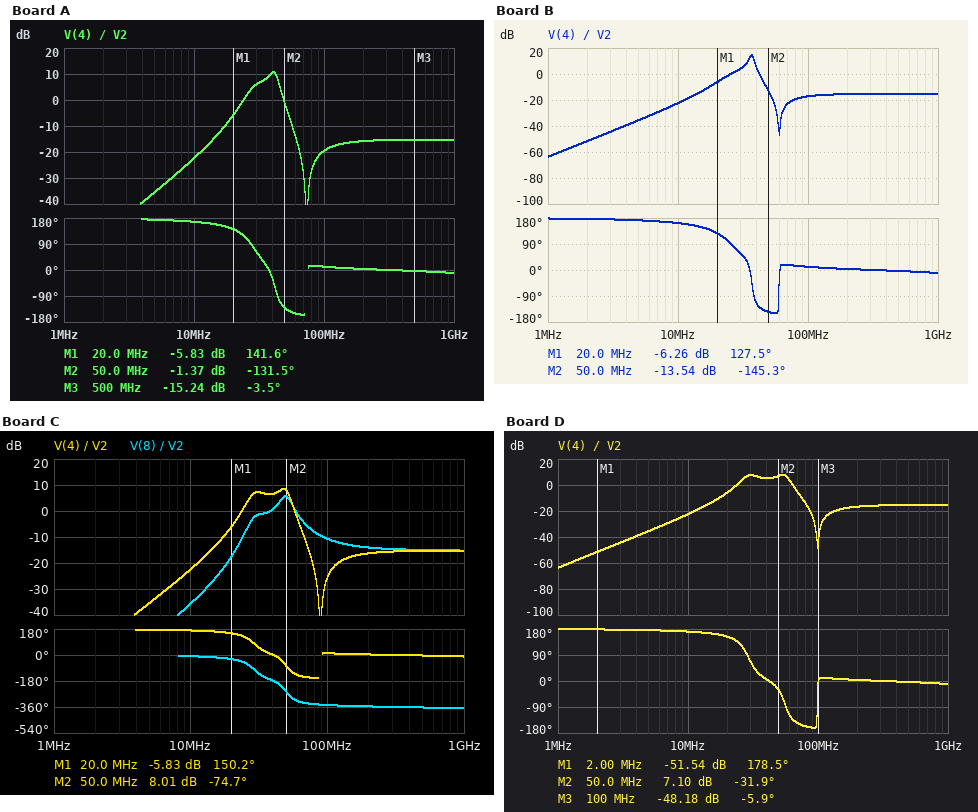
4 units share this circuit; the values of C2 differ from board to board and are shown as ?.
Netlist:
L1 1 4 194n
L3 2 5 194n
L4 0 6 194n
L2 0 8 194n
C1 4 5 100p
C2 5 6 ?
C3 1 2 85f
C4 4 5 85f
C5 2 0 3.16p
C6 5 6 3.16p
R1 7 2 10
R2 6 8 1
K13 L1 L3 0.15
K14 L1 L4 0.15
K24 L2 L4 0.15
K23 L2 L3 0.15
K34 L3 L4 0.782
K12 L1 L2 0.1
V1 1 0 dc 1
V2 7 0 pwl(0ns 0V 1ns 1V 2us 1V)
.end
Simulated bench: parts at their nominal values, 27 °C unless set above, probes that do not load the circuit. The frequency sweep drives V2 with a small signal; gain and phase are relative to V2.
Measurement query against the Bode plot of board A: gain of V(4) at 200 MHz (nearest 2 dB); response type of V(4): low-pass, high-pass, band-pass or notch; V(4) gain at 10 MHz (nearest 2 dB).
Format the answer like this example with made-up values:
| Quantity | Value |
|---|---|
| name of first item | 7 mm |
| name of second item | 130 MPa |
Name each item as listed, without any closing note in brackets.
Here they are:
| Quantity | Value |
|---|---|
| gain of V(4) at 200 MHz | -16 dB |
| response type of V(4): low-pass, high-pass, band-pass or notch | band-pass |
| V(4) gain at 10 MHz | -22 dB |
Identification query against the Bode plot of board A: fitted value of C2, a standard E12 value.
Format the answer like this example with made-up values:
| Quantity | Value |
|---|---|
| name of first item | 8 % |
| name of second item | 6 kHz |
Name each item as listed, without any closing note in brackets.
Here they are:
| Quantity | Value |
|---|---|
| fitted value of C2, a standard E12 value | 220 pF |
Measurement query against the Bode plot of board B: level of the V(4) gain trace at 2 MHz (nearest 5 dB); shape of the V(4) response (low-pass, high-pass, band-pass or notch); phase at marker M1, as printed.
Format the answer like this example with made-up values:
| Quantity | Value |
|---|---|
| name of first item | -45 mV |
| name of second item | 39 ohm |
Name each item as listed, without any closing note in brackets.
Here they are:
| Quantity | Value |
|---|---|
| level of the V(4) gain trace at 2 MHz | -50 dB |
| shape of the V(4) response | band-pass |
| phase at marker M1, as printed | 127.5 deg |
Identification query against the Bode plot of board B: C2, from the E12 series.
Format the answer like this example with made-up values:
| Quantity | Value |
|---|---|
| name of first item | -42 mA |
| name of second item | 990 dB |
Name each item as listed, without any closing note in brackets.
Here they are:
| Quantity | Value |
|---|---|
| C2, from the E12 series | 330 pF |
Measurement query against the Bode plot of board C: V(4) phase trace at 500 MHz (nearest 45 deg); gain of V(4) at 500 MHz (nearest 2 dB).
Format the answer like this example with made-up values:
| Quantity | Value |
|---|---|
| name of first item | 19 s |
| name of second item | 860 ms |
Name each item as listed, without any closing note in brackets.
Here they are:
| Quantity | Value |
|---|---|
| V(4) phase trace at 500 MHz | 0 deg |
| gain of V(4) at 500 MHz | -16 dB |
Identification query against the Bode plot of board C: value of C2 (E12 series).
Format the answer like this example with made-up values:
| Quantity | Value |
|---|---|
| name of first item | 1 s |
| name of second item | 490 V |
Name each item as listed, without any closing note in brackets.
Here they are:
| Quantity | Value |
|---|---|
| value of C2 | 150 pF |
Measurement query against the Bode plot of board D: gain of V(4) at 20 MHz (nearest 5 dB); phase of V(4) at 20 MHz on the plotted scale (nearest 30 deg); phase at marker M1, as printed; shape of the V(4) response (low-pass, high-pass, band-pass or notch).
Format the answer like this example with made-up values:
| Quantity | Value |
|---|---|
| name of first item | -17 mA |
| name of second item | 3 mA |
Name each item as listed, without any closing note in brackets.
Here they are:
| Quantity | Value |
|---|---|
| gain of V(4) at 20 MHz | -5 dB |
| phase of V(4) at 20 MHz on the plotted scale | 150 deg |
| phase at marker M1, as printed | 178.5 deg |
| shape of the V(4) response | band-pass |
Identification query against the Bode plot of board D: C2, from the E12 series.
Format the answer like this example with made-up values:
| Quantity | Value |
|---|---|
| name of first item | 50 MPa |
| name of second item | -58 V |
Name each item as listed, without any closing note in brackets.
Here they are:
| Quantity | Value |
|---|---|
| C2, from the E12 series | 120 pF |
